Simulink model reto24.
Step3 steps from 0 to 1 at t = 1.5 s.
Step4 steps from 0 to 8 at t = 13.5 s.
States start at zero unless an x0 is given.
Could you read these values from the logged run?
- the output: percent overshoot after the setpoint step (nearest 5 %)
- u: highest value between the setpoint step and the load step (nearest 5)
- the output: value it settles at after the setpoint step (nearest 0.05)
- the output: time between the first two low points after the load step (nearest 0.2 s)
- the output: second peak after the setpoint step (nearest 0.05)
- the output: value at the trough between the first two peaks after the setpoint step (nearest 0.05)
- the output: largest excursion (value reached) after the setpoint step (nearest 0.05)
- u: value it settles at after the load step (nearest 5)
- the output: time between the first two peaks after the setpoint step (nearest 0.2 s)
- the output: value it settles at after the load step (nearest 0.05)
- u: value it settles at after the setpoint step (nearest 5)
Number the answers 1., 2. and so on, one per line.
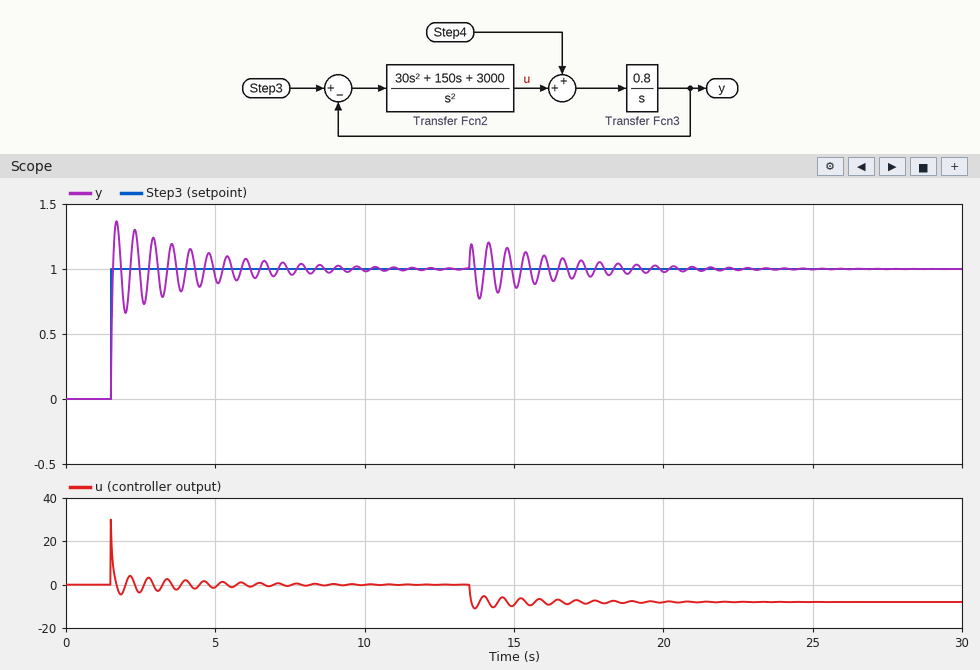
1. 35 %
2. 30
3. 1.00
4. 0.6 s
5. 1.30
6. 0.65
7. 1.35
8. -10
9. 0.6 s
10. 1.00
11. 0
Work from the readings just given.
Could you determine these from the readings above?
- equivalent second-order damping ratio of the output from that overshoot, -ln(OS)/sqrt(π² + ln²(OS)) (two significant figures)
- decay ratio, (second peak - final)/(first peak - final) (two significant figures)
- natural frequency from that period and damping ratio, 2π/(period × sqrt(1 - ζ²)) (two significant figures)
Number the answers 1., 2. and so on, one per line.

1. 0.32
2. 0.86
3. 11 rad/s
